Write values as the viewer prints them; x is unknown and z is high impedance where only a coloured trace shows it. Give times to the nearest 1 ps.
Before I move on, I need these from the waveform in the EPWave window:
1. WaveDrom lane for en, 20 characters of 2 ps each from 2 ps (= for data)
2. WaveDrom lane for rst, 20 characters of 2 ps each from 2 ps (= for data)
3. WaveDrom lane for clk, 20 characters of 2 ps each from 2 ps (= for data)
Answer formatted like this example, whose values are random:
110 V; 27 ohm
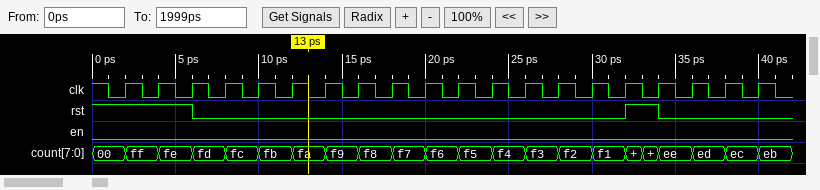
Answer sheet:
{name: 'en', wave: '0...................'}; {name: 'rst', wave: '1.0............10...'}; {name: 'clk', wave: 'p...................'}
